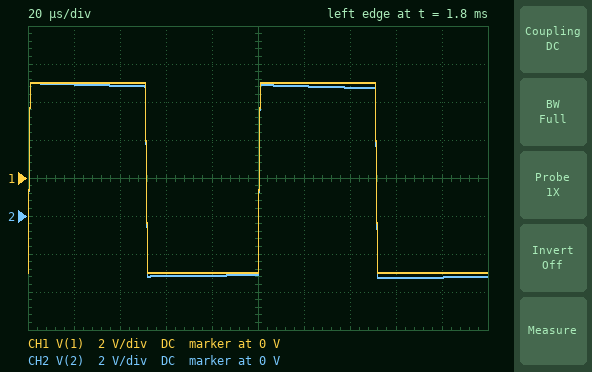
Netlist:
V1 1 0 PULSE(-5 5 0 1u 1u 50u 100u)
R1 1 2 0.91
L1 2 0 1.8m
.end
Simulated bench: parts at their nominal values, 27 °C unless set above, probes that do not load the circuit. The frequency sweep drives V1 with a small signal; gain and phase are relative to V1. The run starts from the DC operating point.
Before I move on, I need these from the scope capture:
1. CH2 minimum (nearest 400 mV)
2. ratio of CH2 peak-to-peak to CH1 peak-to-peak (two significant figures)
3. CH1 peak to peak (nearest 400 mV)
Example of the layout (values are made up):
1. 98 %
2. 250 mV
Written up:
1. -3.2 V
2. 1.0
3. 10.0 V
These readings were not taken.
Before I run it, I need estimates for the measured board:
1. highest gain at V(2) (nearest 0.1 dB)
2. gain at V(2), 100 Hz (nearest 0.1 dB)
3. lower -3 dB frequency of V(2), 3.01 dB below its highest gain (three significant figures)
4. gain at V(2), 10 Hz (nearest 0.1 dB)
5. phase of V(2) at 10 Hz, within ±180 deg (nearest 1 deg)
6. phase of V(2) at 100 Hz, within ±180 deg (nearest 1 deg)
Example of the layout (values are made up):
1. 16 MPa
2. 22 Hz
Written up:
1. 0 dB
2. -2.2 dB
3. 80.5 Hz
4. -18.2 dB
5. 83 deg
6. 39 deg
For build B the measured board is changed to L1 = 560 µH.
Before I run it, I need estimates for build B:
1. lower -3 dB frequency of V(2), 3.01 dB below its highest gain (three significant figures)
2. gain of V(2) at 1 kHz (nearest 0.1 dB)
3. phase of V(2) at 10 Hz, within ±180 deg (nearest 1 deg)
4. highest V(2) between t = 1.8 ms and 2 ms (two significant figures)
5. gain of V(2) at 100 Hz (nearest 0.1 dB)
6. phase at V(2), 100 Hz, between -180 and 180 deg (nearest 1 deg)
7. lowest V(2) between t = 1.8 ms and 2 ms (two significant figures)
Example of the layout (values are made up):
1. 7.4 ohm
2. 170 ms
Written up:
1. 259 Hz
2. -0.3 dB
3. 88 deg
4. 5.4 V
5. -8.9 dB
6. 69 deg
7. -5.1 V
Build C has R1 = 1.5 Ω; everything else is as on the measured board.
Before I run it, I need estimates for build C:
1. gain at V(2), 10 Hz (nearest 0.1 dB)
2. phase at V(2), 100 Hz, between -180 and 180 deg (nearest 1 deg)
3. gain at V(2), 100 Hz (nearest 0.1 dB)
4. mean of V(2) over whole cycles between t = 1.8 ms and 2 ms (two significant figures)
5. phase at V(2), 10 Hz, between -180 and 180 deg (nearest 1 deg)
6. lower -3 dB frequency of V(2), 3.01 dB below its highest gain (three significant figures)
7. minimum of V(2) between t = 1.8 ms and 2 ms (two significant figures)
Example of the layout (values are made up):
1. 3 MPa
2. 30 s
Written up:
1. -22.5 dB
2. 53 deg
3. -4.4 dB
4. 1.0 V
5. 86 deg
6. 133 Hz
7. -4.2 V
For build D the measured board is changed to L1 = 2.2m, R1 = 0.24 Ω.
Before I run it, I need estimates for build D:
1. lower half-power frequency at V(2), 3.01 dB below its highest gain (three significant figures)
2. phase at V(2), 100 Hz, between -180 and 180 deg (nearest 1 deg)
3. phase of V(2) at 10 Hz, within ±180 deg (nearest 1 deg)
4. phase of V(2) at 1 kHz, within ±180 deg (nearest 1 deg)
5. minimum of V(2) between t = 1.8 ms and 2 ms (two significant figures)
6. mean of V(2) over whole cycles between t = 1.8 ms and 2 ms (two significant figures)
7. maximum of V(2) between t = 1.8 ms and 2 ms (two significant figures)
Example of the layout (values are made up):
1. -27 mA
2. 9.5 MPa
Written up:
1. 17.4 Hz
2. 10 deg
3. 60 deg
4. 1 deg
5. -1.0 V
6. 4.1 V
7. 9.1 V
